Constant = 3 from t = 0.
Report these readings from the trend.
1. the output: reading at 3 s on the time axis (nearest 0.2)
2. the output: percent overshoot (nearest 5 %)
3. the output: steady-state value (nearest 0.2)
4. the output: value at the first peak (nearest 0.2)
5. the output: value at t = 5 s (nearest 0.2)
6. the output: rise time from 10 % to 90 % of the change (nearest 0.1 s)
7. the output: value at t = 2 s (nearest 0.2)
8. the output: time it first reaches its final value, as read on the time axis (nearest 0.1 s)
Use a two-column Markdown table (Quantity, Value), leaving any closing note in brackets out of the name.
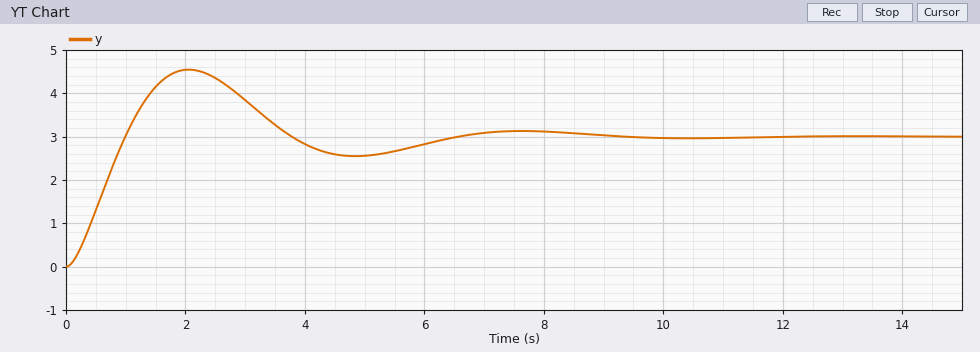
| Quantity | Value |
|---|---|
| the output: reading at 3 s on the time axis | 3.8 |
| the output: percent overshoot | 50 % |
| the output: steady-state value | 3.0 |
| the output: value at the first peak | 4.6 |
| the output: value at t = 5 s | 2.6 |
| the output: rise time from 10 % to 90 % of the change | 0.7 s |
| the output: value at t = 2 s | 4.6 |
| the output: time it first reaches its final value, as read on the time axis | 1.0 s |
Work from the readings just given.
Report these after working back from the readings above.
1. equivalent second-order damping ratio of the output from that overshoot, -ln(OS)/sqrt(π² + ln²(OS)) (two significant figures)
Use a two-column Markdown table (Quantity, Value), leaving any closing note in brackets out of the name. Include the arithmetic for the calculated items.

| Quantity | Value |
|---|---|
| equivalent second-order damping ratio of the output from that overshoot, -ln(OS)/sqrt(π² + ln²(OS)) | ln(0.5) = -0.693; 0.693 / sqrt(9.870 + 0.480) = 0.22 |
